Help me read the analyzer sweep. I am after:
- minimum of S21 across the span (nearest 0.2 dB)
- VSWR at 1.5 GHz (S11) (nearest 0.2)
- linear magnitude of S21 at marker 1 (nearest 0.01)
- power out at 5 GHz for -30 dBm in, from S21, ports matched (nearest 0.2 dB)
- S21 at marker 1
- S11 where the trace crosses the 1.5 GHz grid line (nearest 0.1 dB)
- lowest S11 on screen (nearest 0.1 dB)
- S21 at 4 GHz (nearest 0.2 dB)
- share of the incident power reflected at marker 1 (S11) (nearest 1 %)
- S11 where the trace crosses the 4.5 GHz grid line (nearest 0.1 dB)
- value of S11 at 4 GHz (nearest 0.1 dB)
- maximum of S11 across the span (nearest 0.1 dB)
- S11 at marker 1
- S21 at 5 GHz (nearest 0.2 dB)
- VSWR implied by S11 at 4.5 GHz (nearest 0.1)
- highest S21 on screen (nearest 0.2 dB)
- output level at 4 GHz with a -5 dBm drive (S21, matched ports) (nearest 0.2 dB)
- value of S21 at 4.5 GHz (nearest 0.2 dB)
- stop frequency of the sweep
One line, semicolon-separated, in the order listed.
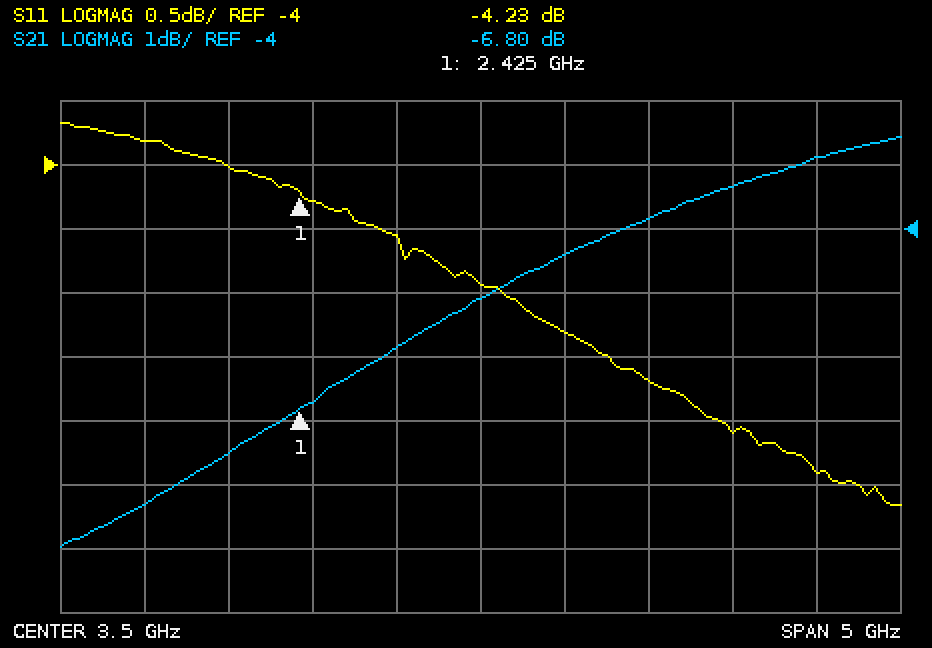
-9.0 dB; 4.6; 0.46; -33.4 dBm; -6.80 dB; -3.8 dB; -6.7 dB; -4.4 dB; 38 %; -5.7 dB; -5.3 dB; -3.7 dB; -4.23 dB; -3.4 dB; 3.2; -2.6 dB; -9.4 dBm; -3.8 dB; 6 GHz
